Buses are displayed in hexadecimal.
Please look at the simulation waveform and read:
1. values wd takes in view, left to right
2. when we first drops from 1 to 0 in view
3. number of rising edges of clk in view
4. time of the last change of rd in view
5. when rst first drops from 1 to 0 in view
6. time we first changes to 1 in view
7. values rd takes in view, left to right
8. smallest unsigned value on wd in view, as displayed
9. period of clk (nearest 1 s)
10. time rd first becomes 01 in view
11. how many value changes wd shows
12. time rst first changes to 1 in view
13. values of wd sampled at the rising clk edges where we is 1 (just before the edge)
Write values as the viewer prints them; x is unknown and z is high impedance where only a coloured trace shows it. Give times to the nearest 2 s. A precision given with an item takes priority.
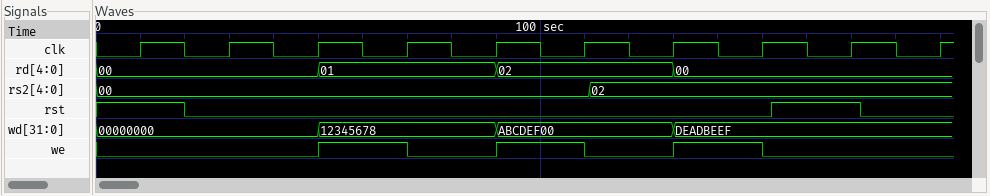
00000000, 12345678, ABCDEF00, DEADBEEF
70 s
10
130 s
20 s
50 s
00, 01, 02, 00
00000000
20 s
50 s
3
152 s
12345678, ABCDEF00, DEADBEEF
